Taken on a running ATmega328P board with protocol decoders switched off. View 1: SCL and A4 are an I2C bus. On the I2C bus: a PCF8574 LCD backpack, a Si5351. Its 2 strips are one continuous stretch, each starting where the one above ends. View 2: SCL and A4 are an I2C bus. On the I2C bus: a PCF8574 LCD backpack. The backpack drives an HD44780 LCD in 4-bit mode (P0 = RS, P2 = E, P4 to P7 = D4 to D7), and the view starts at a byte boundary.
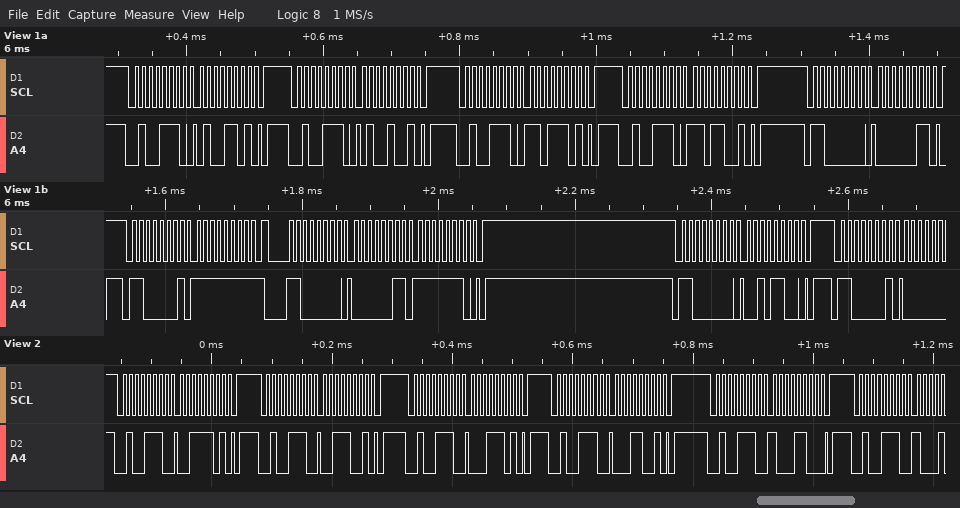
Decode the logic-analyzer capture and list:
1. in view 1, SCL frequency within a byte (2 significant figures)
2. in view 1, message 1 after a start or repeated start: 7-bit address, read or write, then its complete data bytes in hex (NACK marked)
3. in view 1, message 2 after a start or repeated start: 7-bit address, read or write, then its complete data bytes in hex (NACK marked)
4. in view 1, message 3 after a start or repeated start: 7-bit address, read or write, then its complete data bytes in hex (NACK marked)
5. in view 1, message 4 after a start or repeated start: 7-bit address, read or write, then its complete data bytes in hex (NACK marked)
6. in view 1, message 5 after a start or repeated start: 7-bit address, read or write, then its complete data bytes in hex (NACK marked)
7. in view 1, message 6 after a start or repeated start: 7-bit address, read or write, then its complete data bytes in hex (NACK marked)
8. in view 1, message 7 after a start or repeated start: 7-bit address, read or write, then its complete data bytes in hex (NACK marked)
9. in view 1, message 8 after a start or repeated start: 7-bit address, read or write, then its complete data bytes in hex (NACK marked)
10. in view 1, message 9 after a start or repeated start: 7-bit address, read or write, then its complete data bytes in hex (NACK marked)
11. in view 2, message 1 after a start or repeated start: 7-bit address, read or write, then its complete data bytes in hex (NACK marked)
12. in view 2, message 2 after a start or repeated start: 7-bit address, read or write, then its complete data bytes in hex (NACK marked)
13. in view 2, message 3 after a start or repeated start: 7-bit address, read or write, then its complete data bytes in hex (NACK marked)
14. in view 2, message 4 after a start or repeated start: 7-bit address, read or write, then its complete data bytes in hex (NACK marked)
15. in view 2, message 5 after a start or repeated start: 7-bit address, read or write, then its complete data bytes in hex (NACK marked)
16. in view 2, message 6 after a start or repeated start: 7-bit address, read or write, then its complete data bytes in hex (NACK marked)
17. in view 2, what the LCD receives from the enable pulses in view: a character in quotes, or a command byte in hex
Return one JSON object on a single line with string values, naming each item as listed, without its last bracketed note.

{"in view 1, SCL frequency within a byte": "100 kHz", "in view 1, message 1 after a start or repeated start: 7-bit address, read or write, then its complete data bytes in hex": "0x27 write: 4D", "in view 1, message 2 after a start or repeated start: 7-bit address, read or write, then its complete data bytes in hex": "0x27 write: 49", "in view 1, message 3 after a start or repeated start: 7-bit address, read or write, then its complete data bytes in hex": "0x27 write: DD", "in view 1, message 4 after a start or repeated start: 7-bit address, read or write, then its complete data bytes in hex": "0x27 write: D9", "in view 1, message 5 after a start or repeated start: 7-bit address, read or write, then its complete data bytes in hex": "0x60 write: 03", "in view 1, message 6 after a start or repeated start: 7-bit address, read or write, then its complete data bytes in hex": "0x60 read: FF NACK", "in view 1, message 7 after a start or repeated start: 7-bit address, read or write, then its complete data bytes in hex": "0x60 write: 03 FE", "in view 1, message 8 after a start or repeated start: 7-bit address, read or write, then its complete data bytes in hex": "0x60 write: 2C", "in view 1, message 9 after a start or repeated start: 7-bit address, read or write, then its complete data bytes in hex": "0x60 read", "in view 2, message 1 after a start or repeated start: 7-bit address, read or write, then its complete data bytes in hex": "0x27 write: 3D", "in view 2, message 2 after a start or repeated start: 7-bit address, read or write, then its complete data bytes in hex": "0x27 write: 39", "in view 2, message 3 after a start or repeated start: 7-bit address, read or write, then its complete data bytes in hex": "0x27 write: 1D", "in view 2, message 4 after a start or repeated start: 7-bit address, read or write, then its complete data bytes in hex": "0x27 write: 19", "in view 2, message 5 after a start or repeated start: 7-bit address, read or write, then its complete data bytes in hex": "0x27 write: 8C", "in view 2, message 6 after a start or repeated start: 7-bit address, read or write, then its complete data bytes in hex": "0x27 write", "in view 2, what the LCD receives from the enable pulses in view: a character in quotes, or a command byte in hex": "'1'"}
